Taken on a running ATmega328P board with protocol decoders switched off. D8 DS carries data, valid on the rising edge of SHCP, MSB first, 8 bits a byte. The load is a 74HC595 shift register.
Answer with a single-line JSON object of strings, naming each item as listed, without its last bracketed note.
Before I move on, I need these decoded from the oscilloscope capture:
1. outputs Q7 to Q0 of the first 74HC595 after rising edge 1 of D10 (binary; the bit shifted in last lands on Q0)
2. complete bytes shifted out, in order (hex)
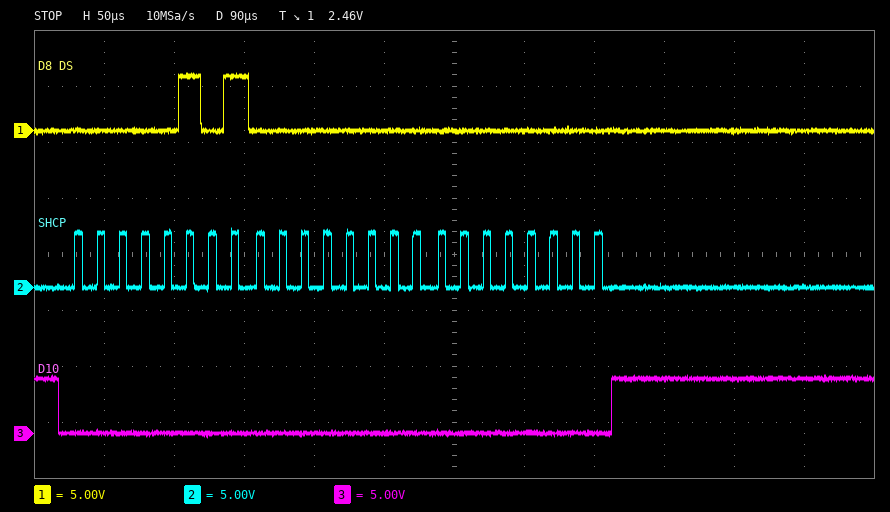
{"outputs Q7 to Q0 of the first 74HC595 after rising edge 1 of D10": "00000000", "complete bytes shifted out, in order": "0x05 0x00 0x00"}
